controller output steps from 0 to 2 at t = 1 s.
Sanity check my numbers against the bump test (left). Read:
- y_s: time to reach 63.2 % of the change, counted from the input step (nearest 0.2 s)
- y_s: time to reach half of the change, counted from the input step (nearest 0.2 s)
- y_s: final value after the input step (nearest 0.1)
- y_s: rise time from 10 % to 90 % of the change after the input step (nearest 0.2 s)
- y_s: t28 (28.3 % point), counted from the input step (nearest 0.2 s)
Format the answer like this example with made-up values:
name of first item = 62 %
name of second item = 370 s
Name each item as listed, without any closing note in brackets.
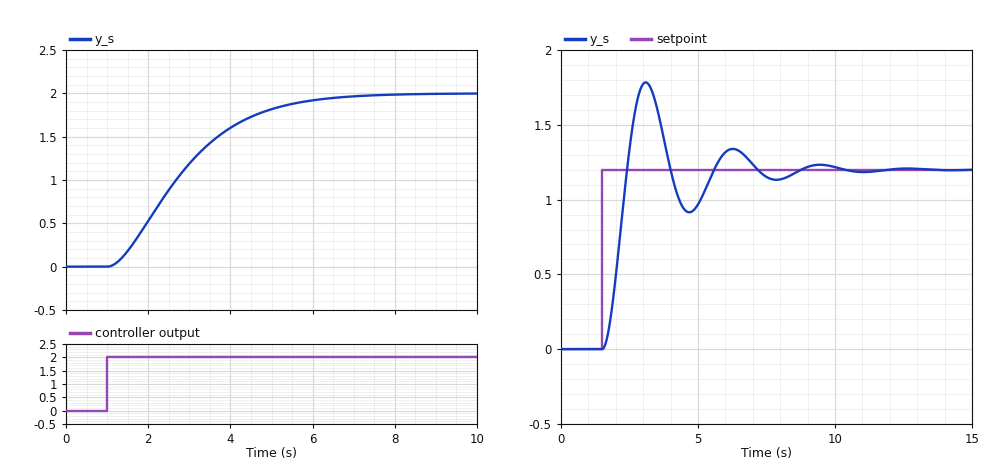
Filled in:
y_s: time to reach 63.2 % of the change, counted from the input step = 2.2 s
y_s: time to reach half of the change, counted from the input step = 1.6 s
y_s: final value after the input step = 2.0
y_s: rise time from 10 % to 90 % of the change after the input step = 3.4 s
y_s: t28 (28.3 % point), counted from the input step = 1.0 s
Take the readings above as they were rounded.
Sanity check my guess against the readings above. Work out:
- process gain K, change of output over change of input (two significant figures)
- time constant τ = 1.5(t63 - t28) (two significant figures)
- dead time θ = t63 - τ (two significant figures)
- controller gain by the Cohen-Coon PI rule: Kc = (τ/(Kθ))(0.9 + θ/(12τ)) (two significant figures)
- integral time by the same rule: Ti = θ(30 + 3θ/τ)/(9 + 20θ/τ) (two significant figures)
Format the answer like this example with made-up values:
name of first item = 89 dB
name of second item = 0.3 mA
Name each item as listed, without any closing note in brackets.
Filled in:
process gain K, change of output over change of input = 1.0
time constant τ = 1.5(t63 - t28) = 1.8 s
dead time θ = t63 - τ = 0.40 s
controller gain by the Cohen-Coon PI rule: Kc = (τ/(Kθ))(0.9 + θ/(12τ)) = 4.1
integral time by the same rule: Ti = θ(30 + 3θ/τ)/(9 + 20θ/τ) = 0.91 s
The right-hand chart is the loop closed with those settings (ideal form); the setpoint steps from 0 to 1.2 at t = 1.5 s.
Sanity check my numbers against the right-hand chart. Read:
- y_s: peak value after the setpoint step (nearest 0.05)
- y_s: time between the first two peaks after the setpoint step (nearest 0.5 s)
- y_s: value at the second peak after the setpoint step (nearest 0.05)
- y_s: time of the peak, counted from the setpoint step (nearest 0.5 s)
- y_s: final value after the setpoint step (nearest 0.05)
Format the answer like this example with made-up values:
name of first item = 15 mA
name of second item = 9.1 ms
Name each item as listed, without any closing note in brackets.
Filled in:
y_s: peak value after the setpoint step = 1.80
y_s: time between the first two peaks after the setpoint step = 3.0 s
y_s: value at the second peak after the setpoint step = 1.35
y_s: time of the peak, counted from the setpoint step = 1.5 s
y_s: final value after the setpoint step = 1.20
